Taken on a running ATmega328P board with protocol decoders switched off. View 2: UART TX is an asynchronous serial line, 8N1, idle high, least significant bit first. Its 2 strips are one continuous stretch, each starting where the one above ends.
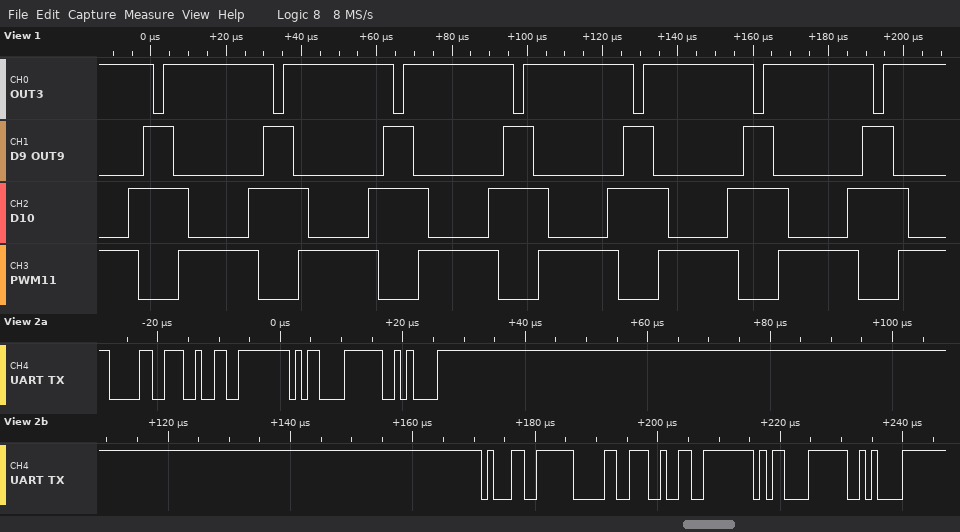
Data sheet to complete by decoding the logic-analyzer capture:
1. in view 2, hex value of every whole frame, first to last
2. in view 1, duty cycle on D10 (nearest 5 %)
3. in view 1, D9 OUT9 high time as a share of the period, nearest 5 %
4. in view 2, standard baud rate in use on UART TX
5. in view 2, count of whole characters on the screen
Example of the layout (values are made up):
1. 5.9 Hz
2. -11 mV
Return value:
1. 0x30 0x32 0x0D 0x0A 0x31 0x30 0x32 0x0D 0x0A
2. 50 %
3. 25 %
4. 1000000 baud
5. 9
